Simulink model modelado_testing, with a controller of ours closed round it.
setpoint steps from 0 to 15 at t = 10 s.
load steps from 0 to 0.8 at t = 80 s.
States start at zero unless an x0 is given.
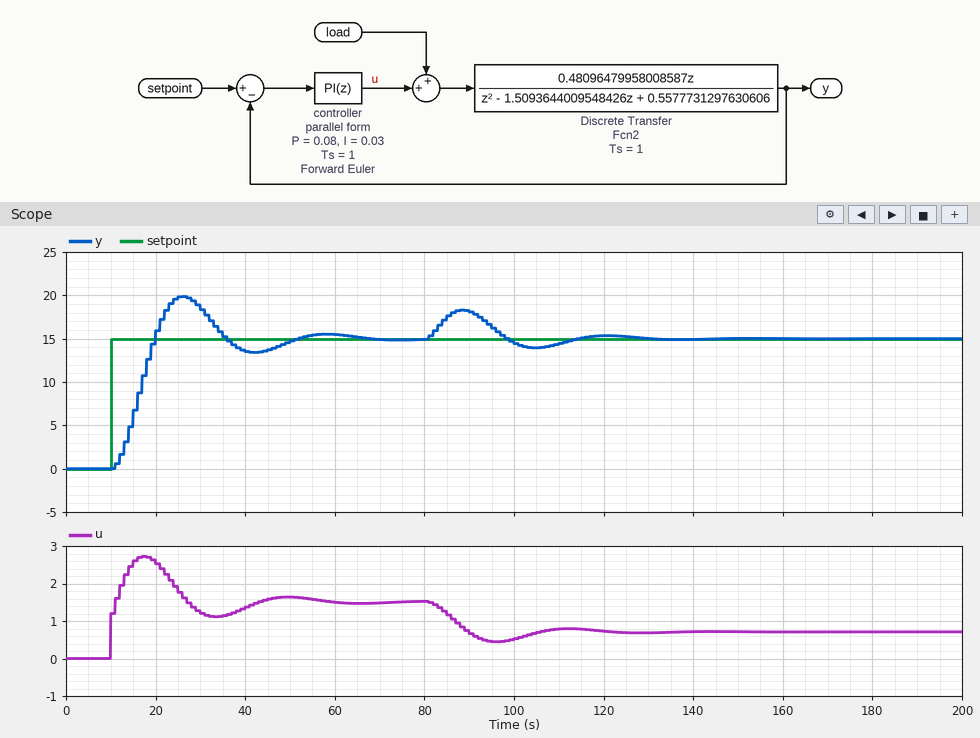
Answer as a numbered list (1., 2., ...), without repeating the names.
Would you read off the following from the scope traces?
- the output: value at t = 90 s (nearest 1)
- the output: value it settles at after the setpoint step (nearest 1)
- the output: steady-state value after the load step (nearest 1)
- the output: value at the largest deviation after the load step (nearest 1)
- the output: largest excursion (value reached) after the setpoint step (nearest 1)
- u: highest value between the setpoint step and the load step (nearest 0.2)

1. 18
2. 15
3. 15
4. 18
5. 20
6. 2.8
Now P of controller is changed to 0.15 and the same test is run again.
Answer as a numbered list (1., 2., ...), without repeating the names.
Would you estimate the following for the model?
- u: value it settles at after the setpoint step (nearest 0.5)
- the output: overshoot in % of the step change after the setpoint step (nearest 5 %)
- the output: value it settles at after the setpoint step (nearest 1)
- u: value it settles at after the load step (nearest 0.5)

1. 1.5
2. 15 %
3. 15
4. 0.5
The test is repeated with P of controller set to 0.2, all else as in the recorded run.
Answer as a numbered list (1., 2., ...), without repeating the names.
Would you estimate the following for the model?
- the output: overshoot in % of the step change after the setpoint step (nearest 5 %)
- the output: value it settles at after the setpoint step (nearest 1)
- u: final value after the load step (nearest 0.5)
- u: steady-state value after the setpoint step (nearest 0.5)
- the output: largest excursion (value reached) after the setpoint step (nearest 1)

1. 10 %
2. 15
3. 0.5
4. 1.5
5. 17
